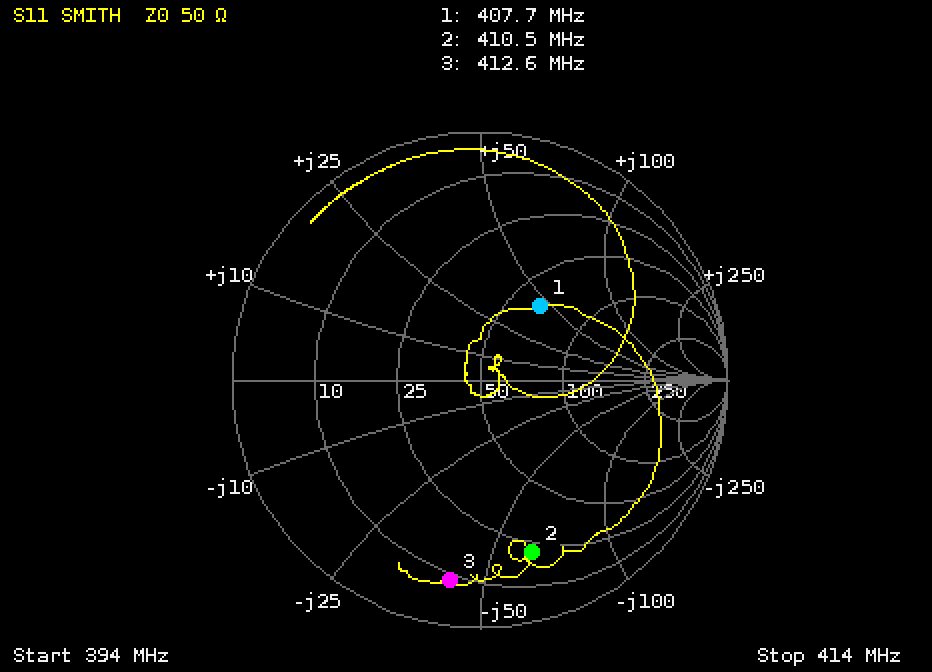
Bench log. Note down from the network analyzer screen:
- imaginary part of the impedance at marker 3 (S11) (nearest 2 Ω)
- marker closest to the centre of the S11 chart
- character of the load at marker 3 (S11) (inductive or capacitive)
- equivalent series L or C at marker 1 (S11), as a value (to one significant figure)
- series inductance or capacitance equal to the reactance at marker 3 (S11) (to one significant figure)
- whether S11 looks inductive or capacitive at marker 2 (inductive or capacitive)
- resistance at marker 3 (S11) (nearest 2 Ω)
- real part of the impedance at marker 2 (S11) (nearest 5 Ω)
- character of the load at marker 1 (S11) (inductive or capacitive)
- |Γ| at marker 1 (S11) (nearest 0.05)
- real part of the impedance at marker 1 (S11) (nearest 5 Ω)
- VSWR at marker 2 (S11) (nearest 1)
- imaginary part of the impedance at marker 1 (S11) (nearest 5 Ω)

-42 Ω
marker 1
capacitive
20 nH
9 pF
capacitive
8 Ω
20 Ω
inductive
0.40
65 Ω
6
+45 Ω
